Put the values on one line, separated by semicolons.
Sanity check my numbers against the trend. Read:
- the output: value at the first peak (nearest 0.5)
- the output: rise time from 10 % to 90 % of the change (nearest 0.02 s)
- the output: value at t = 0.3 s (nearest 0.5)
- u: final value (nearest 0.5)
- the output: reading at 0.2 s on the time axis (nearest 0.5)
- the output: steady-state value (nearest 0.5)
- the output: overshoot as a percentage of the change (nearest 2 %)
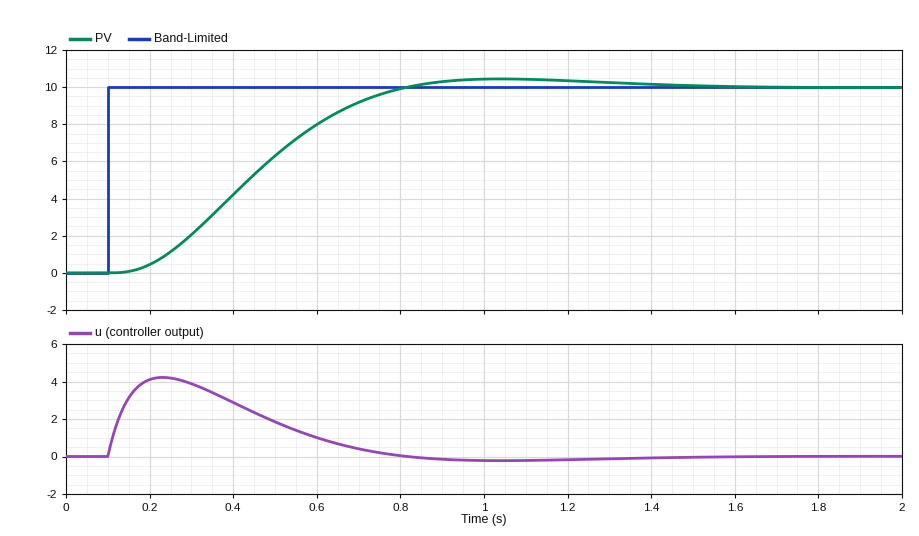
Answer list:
10.5; 0.44 s; 2.0; 0.0; 0.5; 10.0; 4 %
